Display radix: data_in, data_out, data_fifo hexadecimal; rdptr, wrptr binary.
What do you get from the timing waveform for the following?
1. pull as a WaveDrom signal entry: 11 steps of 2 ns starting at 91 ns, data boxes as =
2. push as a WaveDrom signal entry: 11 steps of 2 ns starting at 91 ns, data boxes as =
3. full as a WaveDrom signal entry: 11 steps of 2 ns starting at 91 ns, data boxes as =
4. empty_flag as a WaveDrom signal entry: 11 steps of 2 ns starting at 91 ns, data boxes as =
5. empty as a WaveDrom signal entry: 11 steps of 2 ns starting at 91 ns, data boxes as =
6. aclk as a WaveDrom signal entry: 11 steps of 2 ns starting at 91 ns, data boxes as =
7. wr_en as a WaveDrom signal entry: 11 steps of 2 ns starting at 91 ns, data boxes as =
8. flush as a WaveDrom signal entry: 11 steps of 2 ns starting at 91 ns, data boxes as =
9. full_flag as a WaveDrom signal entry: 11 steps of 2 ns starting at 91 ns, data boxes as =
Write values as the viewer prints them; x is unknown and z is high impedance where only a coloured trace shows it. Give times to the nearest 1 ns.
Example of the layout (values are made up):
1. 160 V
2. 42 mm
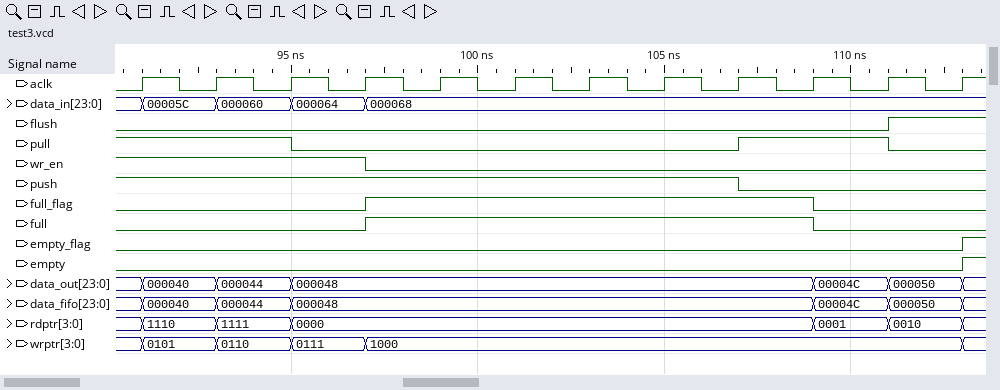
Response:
1. {name: 'pull', wave: '1.0.....1.0'}
2. {name: 'push', wave: '1.......0..'}
3. {name: 'full', wave: '0..1.....0.'}
4. {name: 'empty_flag', wave: '0..........'}
5. {name: 'empty', wave: '0..........'}
6. {name: 'aclk', wave: 'p..........'}
7. {name: 'wr_en', wave: '1..0.......'}
8. {name: 'flush', wave: '0.........1'}
9. {name: 'full_flag', wave: '0..1.....0.'}
